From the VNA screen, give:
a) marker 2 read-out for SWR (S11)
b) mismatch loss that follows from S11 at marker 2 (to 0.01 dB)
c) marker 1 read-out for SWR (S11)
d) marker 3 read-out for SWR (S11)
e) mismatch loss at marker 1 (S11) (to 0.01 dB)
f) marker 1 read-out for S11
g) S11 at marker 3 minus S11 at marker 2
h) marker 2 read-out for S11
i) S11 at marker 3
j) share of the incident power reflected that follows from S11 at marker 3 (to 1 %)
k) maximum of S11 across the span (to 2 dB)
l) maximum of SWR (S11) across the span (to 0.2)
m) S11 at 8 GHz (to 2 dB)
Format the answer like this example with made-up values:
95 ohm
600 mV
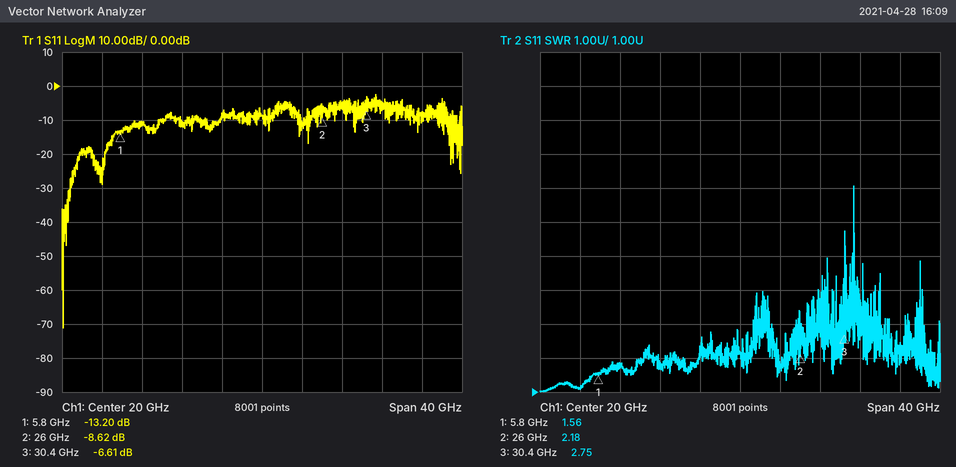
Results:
2.18
0.64 dB
1.56
2.75
0.21 dB
-13.20 dB
2.01 dB
-8.62 dB
-6.61 dB
22 %
-2 dB
7.0
-12 dB
